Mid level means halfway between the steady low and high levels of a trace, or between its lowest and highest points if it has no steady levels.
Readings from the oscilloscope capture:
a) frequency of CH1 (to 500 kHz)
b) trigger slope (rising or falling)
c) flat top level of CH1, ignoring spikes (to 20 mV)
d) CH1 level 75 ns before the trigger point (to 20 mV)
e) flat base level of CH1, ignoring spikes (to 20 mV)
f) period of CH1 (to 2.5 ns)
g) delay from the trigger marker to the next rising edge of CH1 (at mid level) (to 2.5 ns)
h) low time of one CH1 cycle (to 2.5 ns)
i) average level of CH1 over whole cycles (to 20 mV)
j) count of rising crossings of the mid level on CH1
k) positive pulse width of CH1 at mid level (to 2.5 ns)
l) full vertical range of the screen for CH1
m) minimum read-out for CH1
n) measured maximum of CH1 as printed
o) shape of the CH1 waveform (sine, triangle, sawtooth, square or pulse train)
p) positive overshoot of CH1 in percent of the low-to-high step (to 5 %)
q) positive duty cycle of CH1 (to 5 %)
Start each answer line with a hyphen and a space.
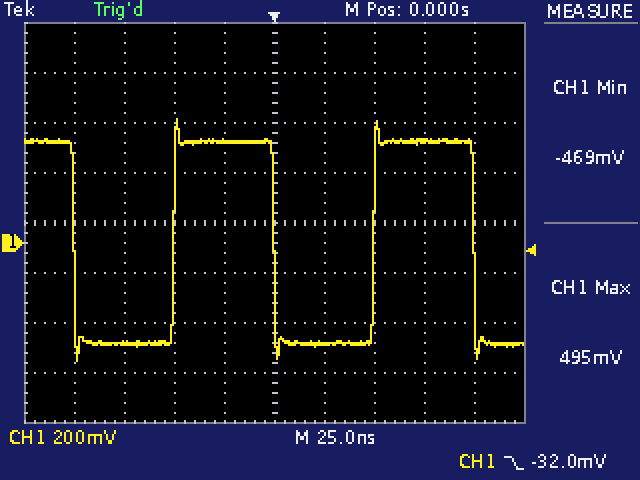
- 10.0 MHz
- falling
- 400 mV
- -400 mV
- -400 mV
- 100.0 ns
- 50.0 ns
- 50.0 ns
- 0 mV
- 2
- 50.0 ns
- 1.6 V
- -469 mV
- 495 mV
- square
- 10 %
- 50 %
